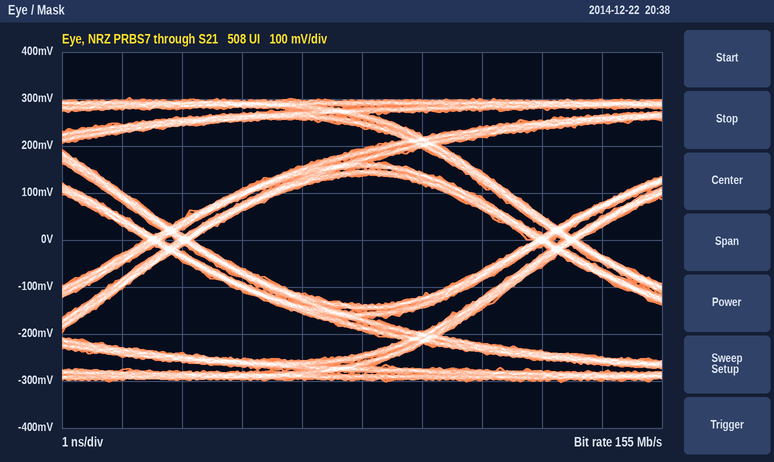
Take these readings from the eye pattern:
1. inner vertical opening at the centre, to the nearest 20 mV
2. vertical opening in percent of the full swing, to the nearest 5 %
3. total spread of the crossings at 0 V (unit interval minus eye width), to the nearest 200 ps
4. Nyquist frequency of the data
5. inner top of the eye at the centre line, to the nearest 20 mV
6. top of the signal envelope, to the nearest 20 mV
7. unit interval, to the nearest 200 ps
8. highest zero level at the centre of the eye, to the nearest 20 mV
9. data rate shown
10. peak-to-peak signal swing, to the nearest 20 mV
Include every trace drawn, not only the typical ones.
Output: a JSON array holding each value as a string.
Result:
["280 mV", "45 %", "800 ps", "77.5 MHz", "140 mV", "300 mV", "6.4 ns", "-140 mV", "155 Mb/s", "600 mV"]
